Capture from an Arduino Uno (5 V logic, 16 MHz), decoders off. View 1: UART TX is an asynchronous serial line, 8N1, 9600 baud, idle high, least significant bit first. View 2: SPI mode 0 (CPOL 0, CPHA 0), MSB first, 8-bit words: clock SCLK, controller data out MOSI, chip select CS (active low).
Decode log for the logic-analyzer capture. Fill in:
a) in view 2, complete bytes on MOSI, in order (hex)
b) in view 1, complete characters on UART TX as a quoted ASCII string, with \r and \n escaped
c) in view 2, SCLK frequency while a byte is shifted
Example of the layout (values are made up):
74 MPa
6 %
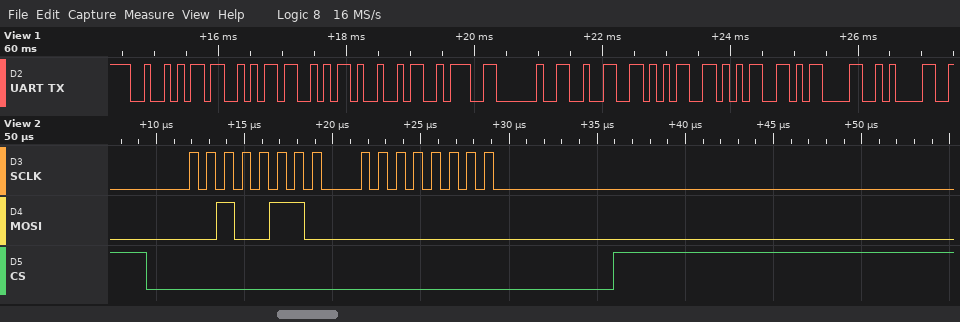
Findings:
0x26 0x00
"RSSI: 255\r\n"
1 MHz
